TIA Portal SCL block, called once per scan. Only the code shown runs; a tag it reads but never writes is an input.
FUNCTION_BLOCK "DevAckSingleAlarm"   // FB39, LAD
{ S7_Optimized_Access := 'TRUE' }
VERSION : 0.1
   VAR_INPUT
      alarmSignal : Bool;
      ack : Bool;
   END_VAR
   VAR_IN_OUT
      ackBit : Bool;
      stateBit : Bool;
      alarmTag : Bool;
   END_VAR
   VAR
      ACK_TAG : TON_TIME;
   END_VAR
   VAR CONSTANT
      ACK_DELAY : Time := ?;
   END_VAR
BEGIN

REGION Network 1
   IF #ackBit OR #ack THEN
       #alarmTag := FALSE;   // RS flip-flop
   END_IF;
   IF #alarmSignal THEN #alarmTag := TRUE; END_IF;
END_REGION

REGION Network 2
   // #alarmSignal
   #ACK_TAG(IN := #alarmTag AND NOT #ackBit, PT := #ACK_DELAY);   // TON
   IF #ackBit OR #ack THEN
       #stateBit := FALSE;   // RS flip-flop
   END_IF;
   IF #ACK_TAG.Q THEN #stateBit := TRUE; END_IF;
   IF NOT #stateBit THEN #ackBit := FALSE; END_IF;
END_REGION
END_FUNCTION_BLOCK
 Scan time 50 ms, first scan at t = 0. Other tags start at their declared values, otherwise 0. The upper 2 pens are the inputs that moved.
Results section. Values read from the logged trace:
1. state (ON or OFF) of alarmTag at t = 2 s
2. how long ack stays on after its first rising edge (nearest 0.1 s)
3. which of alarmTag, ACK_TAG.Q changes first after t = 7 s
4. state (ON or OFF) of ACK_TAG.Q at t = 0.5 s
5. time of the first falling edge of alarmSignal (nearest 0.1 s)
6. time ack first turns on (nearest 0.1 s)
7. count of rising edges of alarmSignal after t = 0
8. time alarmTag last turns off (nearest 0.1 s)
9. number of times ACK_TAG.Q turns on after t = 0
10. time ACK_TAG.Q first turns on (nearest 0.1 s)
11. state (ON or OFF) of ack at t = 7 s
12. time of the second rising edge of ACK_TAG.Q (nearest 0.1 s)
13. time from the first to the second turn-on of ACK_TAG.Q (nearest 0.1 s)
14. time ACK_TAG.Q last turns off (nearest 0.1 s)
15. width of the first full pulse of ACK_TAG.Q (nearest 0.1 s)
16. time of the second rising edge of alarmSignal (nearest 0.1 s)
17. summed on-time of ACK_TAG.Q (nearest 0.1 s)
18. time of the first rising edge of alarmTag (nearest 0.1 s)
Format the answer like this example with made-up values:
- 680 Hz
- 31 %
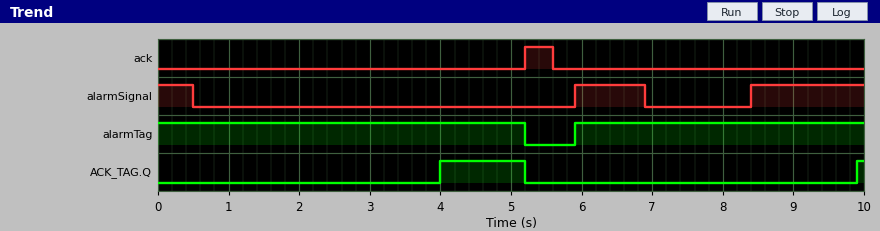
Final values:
- ON
- 0.4 s
- ACK_TAG.Q
- OFF
- 0.5 s
- 5.2 s
- 2
- 5.2 s
- 2
- 4.0 s
- OFF
- 9.9 s
- 5.9 s
- 5.2 s
- 1.2 s
- 8.4 s
- 1.3 s
- 5.9 s
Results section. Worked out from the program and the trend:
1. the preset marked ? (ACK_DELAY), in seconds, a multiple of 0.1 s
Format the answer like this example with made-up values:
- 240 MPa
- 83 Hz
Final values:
- 4.0 s
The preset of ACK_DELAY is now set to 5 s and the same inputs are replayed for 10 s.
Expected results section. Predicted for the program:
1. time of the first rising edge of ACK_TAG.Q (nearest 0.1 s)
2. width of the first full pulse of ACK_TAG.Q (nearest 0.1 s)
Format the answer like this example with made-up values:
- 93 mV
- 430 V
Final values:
- 5.0 s
- 0.2 s
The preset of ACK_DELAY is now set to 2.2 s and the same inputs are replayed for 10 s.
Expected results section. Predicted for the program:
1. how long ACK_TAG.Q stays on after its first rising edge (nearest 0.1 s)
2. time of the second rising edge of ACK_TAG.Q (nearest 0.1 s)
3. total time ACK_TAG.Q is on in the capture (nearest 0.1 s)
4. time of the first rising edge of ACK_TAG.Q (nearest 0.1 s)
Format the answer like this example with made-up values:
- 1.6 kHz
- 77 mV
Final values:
- 3.0 s
- 8.1 s
- 4.9 s
- 2.2 s
